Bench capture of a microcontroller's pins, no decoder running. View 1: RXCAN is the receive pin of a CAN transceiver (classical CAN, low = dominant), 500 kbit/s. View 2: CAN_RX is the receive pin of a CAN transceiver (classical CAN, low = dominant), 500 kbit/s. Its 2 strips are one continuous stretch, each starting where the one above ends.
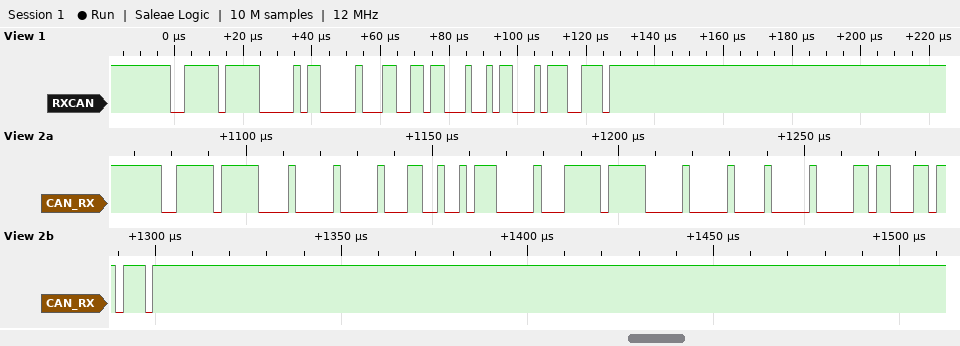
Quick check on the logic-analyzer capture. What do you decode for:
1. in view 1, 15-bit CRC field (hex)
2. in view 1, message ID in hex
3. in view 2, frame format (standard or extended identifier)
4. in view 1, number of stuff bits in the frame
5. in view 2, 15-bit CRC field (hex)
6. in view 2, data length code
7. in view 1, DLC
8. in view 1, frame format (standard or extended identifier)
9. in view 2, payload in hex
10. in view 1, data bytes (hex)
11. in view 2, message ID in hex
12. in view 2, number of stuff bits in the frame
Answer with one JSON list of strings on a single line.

["0x3173", "0x3FF", "standard", "4", "0x58DB", "8", "3", "standard", "00 32 5C 03 FF 00 04 00", "00 CD 89", "0x3FF", "11"]
